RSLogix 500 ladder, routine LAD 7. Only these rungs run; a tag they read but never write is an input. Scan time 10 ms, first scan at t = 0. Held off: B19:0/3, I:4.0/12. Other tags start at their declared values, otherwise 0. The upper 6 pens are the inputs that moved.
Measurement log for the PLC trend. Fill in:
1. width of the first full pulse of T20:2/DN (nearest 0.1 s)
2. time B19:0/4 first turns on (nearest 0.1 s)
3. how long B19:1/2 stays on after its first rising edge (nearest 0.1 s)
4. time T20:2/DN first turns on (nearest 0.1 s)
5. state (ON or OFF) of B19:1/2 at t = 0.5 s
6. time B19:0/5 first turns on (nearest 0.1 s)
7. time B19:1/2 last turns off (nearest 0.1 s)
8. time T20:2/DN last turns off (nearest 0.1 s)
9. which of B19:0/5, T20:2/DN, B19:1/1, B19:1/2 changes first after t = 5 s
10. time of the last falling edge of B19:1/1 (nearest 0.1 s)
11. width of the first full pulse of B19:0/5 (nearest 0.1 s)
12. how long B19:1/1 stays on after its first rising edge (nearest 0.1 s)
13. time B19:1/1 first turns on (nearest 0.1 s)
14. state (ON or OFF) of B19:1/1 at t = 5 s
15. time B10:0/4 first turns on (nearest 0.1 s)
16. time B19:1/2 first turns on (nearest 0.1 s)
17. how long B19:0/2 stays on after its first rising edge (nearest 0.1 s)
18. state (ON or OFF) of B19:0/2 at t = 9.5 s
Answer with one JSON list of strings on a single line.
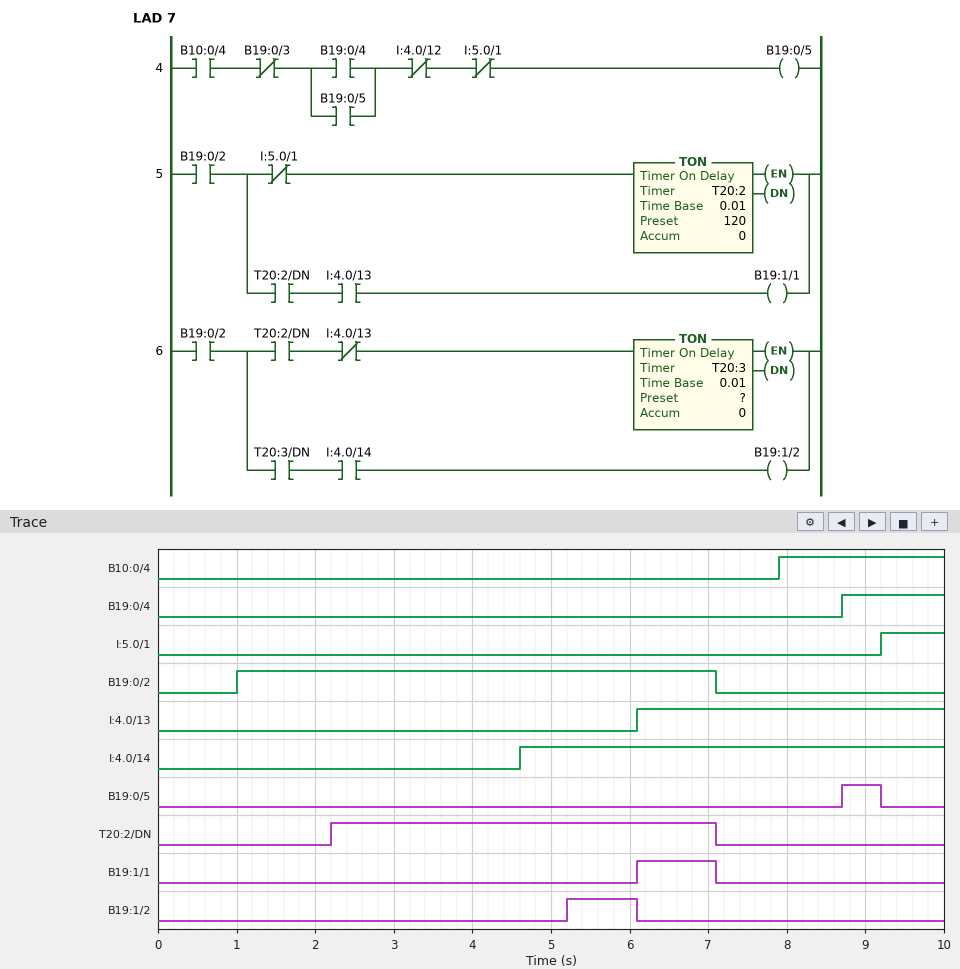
["4.9 s", "8.7 s", "0.9 s", "2.2 s", "OFF", "8.7 s", "6.1 s", "7.1 s", "B19:1/2", "7.1 s", "0.5 s", "1.0 s", "6.1 s", "OFF", "7.9 s", "5.2 s", "6.1 s", "OFF"]
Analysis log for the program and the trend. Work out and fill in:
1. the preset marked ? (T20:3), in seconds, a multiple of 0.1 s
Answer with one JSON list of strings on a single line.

["3.0 s"]
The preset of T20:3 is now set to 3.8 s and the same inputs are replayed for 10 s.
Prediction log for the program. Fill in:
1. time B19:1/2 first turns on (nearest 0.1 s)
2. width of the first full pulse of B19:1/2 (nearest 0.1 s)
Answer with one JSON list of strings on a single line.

["6.0 s", "0.1 s"]
